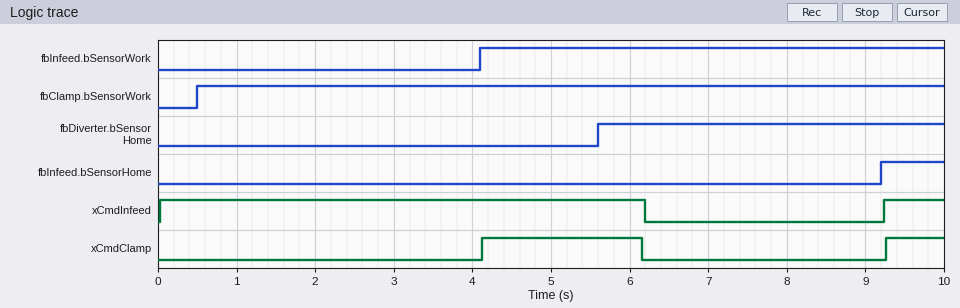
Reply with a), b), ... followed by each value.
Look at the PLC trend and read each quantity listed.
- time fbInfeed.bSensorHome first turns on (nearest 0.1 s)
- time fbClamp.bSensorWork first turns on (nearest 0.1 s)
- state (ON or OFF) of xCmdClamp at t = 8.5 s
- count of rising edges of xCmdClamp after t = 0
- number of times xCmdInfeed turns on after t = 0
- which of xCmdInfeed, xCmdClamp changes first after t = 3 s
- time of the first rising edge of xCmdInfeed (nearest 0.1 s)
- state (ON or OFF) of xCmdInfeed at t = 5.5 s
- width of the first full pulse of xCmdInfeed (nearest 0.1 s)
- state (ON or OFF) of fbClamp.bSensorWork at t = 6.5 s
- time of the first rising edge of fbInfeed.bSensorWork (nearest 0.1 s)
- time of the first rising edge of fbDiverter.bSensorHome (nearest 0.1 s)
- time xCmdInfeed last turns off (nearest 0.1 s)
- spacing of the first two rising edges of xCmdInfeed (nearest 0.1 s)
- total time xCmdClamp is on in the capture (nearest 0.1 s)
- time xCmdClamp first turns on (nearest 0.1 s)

a) 9.2 s
b) 0.5 s
c) OFF
d) 2
e) 2
f) xCmdClamp
g) 0.0 s
h) ON
i) 6.2 s
j) ON
k) 4.1 s
l) 5.6 s
m) 6.2 s
n) 9.2 s
o) 2.8 s
p) 4.1 s
